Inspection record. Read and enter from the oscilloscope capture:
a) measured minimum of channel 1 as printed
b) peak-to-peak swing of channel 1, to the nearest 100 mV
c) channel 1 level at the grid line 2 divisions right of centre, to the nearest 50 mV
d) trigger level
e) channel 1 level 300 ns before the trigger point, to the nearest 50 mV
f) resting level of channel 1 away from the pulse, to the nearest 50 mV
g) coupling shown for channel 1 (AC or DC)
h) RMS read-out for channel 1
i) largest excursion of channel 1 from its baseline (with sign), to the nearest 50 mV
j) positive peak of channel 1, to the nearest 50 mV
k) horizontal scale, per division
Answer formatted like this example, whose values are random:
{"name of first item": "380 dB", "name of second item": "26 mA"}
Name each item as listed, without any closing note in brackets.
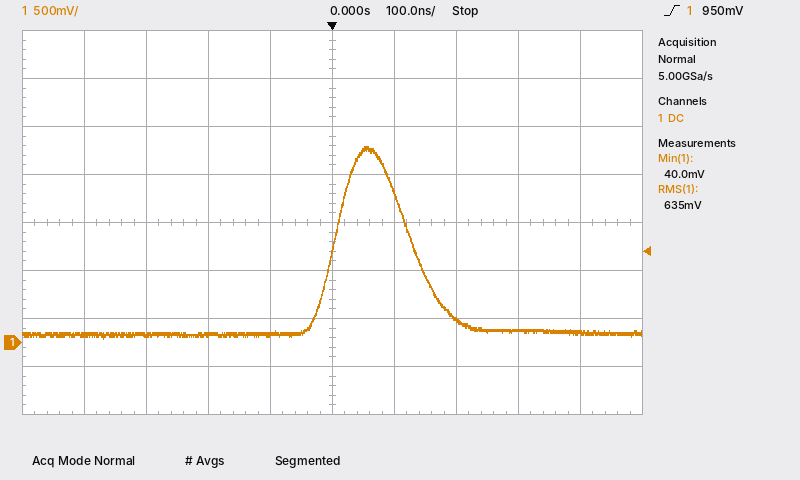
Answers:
{"measured minimum of channel 1 as printed": "40.0 mV", "peak-to-peak swing of channel 1, to the nearest 100 mV": "2.00 V", "channel 1 level at the grid line 2 divisions right of centre, to the nearest 50 mV": "250 mV", "trigger level": "950 mV", "channel 1 level 300 ns before the trigger point, to the nearest 50 mV": "100 mV", "resting level of channel 1 away from the pulse, to the nearest 50 mV": "100 mV", "coupling shown for channel 1": "DC", "RMS read-out for channel 1": "635 mV", "largest excursion of channel 1 from its baseline (with sign), to the nearest 50 mV": "+1.95 V", "positive peak of channel 1, to the nearest 50 mV": "2.05 V", "horizontal scale, per division": "100 ns"}
